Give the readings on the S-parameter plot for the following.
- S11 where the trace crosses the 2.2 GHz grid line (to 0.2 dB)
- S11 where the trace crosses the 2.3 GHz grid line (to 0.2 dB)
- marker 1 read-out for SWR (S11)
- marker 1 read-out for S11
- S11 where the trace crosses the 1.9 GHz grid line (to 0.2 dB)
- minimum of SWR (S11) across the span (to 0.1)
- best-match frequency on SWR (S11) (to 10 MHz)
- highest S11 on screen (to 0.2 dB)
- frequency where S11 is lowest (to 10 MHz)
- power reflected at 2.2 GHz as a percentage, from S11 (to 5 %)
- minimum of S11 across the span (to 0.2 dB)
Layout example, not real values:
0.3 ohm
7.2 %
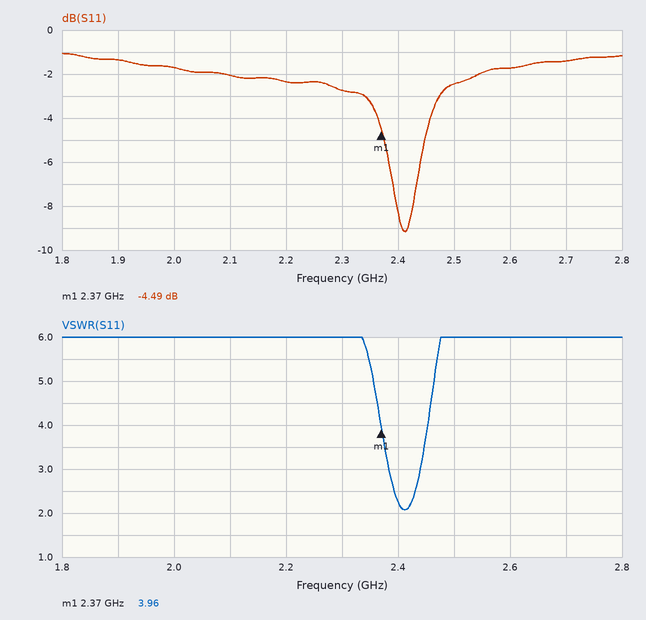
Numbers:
-2.4 dB
-2.8 dB
3.96
-4.49 dB
-1.4 dB
2.1
2.41 GHz
-1.0 dB
2.41 GHz
60 %
-9.2 dB
